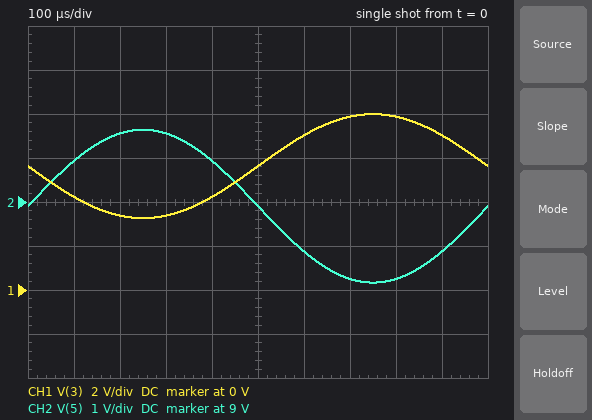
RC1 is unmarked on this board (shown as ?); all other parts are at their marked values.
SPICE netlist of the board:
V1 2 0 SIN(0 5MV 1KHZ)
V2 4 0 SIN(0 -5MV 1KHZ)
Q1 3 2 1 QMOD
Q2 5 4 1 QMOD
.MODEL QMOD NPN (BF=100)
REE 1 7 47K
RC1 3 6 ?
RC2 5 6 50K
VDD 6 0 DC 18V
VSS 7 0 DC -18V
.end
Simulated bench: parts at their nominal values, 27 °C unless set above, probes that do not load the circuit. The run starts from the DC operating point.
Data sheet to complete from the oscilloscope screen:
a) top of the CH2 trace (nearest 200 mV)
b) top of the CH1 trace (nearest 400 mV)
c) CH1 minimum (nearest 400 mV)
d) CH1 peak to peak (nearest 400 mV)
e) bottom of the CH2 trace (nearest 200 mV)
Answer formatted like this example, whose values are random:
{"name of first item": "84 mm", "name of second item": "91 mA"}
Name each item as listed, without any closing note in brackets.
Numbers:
{"top of the CH2 trace": "10.6 V", "top of the CH1 trace": "8.0 V", "CH1 minimum": "3.2 V", "CH1 peak to peak": "4.8 V", "bottom of the CH2 trace": "7.2 V"}
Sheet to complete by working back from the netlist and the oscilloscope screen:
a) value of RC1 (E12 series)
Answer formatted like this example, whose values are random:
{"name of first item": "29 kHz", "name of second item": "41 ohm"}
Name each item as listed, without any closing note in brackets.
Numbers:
{"value of RC1": "68 kΩ"}
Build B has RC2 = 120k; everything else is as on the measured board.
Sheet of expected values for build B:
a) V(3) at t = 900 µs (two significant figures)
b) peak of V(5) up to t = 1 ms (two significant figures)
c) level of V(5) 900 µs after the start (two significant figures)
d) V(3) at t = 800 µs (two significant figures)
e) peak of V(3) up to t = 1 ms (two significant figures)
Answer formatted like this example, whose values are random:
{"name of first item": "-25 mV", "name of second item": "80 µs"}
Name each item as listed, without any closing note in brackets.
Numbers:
{"V(3) at t = 900 µs": "6.1 V", "peak of V(5) up to t = 1 ms": "340 mV", "level of V(5) 900 µs after the start": "-680 mV", "V(3) at t = 800 µs": "6.7 V", "peak of V(3) up to t = 1 ms": "6.8 V"}
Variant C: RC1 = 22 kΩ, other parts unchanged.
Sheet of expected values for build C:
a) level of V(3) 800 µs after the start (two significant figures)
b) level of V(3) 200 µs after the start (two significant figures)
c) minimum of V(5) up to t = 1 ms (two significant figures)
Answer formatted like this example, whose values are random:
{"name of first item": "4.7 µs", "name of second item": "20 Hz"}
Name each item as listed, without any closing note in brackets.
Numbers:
{"level of V(3) 800 µs after the start": "15 V", "level of V(3) 200 µs after the start": "13 V", "minimum of V(5) up to t = 1 ms": "7.2 V"}
